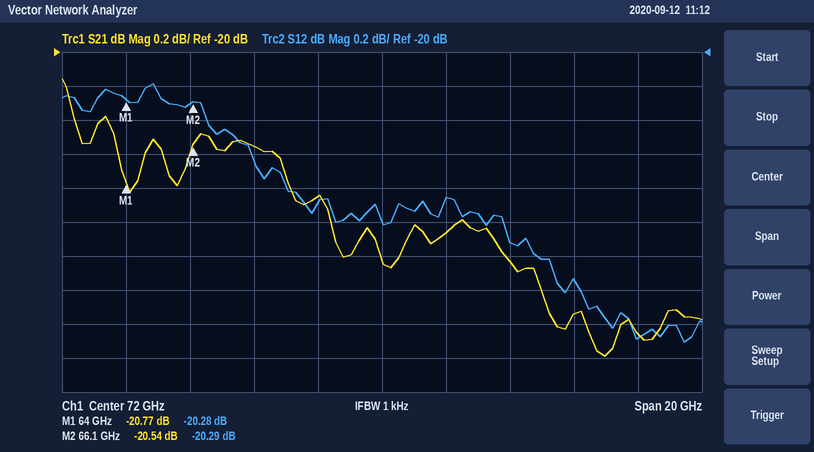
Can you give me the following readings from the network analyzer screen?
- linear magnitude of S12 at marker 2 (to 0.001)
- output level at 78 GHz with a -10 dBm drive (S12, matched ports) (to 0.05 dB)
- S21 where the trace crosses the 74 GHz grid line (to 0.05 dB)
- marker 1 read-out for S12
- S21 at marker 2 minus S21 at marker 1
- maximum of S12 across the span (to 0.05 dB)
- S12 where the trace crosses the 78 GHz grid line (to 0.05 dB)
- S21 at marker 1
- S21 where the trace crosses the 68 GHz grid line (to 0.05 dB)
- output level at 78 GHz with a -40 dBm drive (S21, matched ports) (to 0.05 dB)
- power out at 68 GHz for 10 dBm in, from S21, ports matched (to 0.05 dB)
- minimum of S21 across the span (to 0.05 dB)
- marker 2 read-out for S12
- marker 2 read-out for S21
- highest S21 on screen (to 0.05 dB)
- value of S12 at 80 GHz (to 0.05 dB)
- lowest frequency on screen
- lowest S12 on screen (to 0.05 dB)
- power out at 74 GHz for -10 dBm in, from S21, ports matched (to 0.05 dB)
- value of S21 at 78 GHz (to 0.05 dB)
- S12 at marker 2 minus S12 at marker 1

0.097
-31.35 dBm
-21.05 dB
-20.28 dB
0.23 dB
-20.20 dB
-21.35 dB
-20.77 dB
-20.55 dB
-61.55 dBm
-10.55 dBm
-21.80 dB
-20.29 dB
-20.54 dB
-20.15 dB
-21.70 dB
62 GHz
-21.70 dB
-31.05 dBm
-21.55 dB
-0.01 dB
